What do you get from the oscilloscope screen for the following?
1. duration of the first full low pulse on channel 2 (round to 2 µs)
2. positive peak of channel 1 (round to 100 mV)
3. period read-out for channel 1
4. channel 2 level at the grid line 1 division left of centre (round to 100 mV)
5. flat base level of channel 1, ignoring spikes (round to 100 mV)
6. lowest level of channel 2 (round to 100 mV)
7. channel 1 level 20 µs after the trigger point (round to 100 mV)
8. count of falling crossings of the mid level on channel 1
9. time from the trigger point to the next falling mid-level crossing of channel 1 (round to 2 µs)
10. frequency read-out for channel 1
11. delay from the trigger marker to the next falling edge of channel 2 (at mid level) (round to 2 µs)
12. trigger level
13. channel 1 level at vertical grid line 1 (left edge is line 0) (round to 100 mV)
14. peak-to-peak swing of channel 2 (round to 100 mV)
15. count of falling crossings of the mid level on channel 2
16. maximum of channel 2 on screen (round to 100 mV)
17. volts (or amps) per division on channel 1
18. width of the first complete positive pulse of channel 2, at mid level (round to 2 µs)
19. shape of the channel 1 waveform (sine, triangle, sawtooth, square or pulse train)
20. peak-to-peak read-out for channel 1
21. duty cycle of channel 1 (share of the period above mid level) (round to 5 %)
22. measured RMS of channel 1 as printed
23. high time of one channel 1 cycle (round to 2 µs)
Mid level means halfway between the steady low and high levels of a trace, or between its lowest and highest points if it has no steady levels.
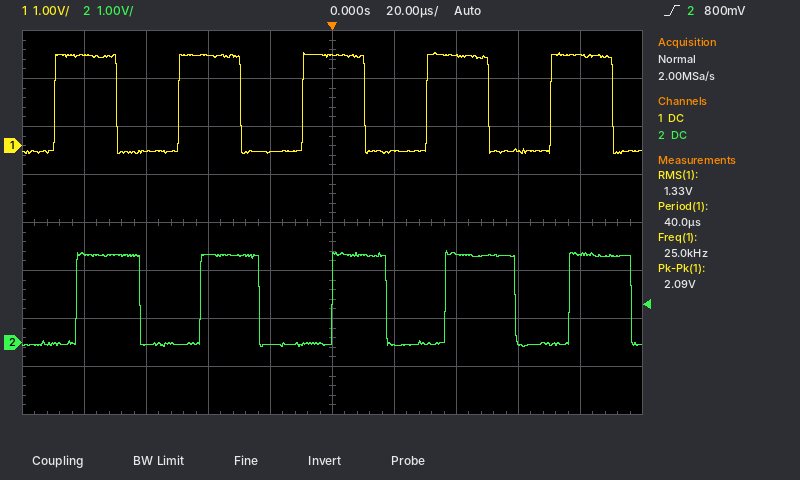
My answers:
20 µs
1.9 V
40.0 µs
0.0 V
-100 mV
-100 mV
-100 mV
5
10 µs
25.0 kHz
18 µs
800 mV
1.9 V
2.0 V
5
1.9 V
1 V
20 µs
square
2.09 V
50 %
1.33 V
20 µs
